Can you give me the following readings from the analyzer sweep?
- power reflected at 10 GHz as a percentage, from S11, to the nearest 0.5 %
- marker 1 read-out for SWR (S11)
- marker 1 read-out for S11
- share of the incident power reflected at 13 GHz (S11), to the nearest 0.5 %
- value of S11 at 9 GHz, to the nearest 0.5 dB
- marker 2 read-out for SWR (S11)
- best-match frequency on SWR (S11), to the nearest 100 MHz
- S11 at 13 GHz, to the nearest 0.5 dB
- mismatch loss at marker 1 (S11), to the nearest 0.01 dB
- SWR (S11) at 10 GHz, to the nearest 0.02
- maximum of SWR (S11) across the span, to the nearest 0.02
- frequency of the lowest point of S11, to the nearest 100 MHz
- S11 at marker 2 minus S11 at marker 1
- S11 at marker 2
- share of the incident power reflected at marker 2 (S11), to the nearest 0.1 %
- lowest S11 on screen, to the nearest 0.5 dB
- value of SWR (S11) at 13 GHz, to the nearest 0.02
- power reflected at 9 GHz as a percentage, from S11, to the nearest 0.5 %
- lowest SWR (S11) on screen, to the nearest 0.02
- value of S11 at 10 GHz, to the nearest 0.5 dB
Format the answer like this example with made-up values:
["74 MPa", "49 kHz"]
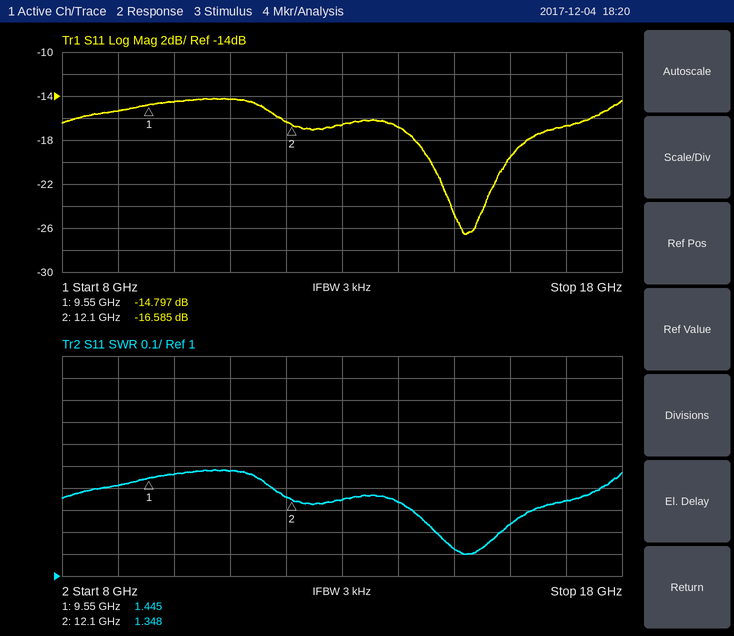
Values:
["3.5 %", "1.445", "-14.797 dB", "2.0 %", "-15.5 dB", "1.348", "15.2 GHz", "-16.5 dB", "0.15 dB", "1.46", "1.48", "15.2 GHz", "-1.788 dB", "-16.585 dB", "2.2 %", "-26.5 dB", "1.34", "3.0 %", "1.10", "-14.5 dB"]
